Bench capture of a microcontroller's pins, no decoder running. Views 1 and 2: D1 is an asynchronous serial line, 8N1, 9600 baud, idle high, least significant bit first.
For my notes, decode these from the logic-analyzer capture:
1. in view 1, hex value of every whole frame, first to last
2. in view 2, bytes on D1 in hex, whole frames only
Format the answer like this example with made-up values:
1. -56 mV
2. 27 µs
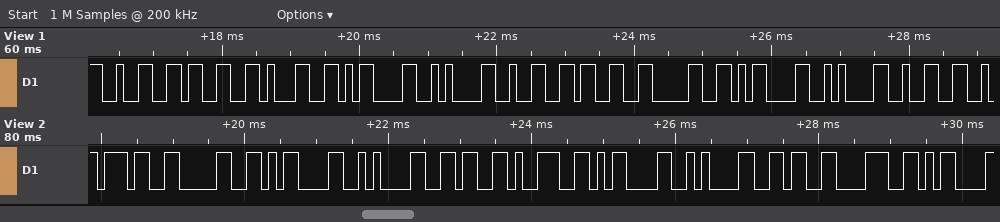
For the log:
1. 32 33 31 0D 0A 32 33 30 0D 0A 32
2. 37 30 0D 0A 36 39 0D 0A 36 38 0D
